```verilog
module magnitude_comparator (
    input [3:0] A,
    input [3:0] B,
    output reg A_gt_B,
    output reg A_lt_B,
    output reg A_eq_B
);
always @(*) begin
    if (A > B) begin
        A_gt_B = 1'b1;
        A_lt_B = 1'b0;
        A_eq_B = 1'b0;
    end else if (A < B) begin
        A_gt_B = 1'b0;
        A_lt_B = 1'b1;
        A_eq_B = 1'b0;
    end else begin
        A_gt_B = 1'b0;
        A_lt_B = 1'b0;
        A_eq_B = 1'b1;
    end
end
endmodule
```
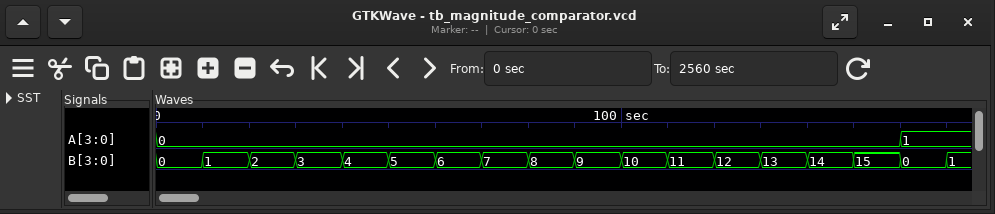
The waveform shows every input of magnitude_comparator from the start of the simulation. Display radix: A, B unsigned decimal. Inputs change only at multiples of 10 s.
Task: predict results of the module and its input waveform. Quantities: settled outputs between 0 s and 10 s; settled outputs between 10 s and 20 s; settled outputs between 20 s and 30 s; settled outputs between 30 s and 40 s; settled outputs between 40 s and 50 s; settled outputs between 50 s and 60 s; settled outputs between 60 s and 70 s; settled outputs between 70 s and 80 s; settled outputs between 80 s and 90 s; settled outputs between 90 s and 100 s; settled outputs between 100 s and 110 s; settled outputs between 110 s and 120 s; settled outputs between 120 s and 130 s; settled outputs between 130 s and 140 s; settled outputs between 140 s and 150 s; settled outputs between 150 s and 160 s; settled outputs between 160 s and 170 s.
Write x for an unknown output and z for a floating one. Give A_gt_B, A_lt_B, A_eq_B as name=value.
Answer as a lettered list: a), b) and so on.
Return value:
a) A_gt_B=0, A_lt_B=0, A_eq_B=1
b) A_gt_B=0, A_lt_B=1, A_eq_B=0
c) A_gt_B=0, A_lt_B=1, A_eq_B=0
d) A_gt_B=0, A_lt_B=1, A_eq_B=0
e) A_gt_B=0, A_lt_B=1, A_eq_B=0
f) A_gt_B=0, A_lt_B=1, A_eq_B=0
g) A_gt_B=0, A_lt_B=1, A_eq_B=0
h) A_gt_B=0, A_lt_B=1, A_eq_B=0
i) A_gt_B=0, A_lt_B=1, A_eq_B=0
j) A_gt_B=0, A_lt_B=1, A_eq_B=0
k) A_gt_B=0, A_lt_B=1, A_eq_B=0
l) A_gt_B=0, A_lt_B=1, A_eq_B=0
m) A_gt_B=0, A_lt_B=1, A_eq_B=0
n) A_gt_B=0, A_lt_B=1, A_eq_B=0
o) A_gt_B=0, A_lt_B=1, A_eq_B=0
p) A_gt_B=0, A_lt_B=1, A_eq_B=0
q) A_gt_B=1, A_lt_B=0, A_eq_B=0
